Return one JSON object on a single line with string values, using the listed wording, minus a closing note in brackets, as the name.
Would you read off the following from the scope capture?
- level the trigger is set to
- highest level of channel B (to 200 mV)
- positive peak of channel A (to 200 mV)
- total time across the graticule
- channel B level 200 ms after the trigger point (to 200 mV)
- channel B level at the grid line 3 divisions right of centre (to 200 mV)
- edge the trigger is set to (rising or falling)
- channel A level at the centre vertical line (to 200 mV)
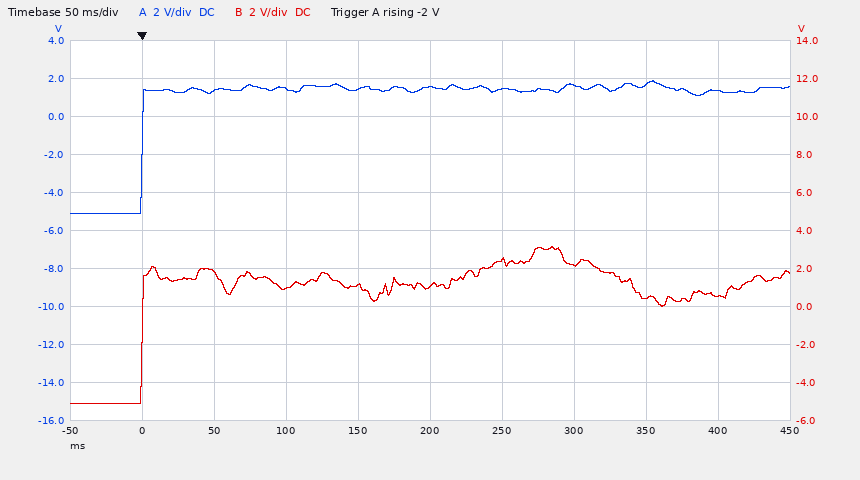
{"level the trigger is set to": "-2 V", "highest level of channel B": "3.2 V", "positive peak of channel A": "1.8 V", "total time across the graticule": "500 ms", "channel B level 200 ms after the trigger point": "1.0 V", "channel B level at the grid line 3 divisions right of centre": "400 mV", "edge the trigger is set to": "rising", "channel A level at the centre vertical line": "1.6 V"}
